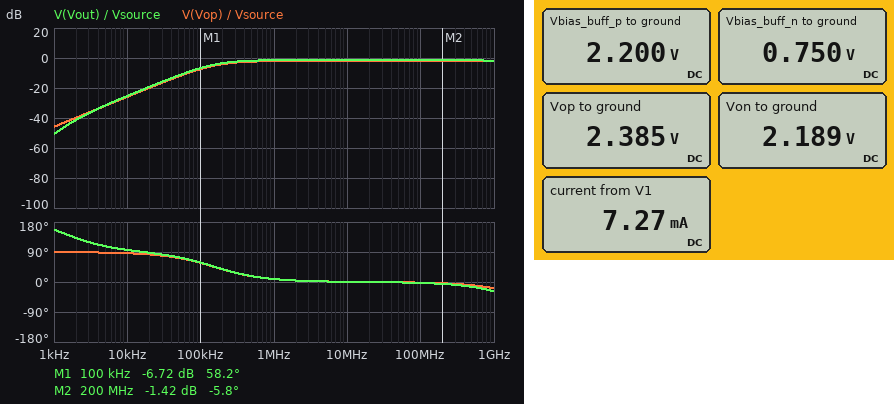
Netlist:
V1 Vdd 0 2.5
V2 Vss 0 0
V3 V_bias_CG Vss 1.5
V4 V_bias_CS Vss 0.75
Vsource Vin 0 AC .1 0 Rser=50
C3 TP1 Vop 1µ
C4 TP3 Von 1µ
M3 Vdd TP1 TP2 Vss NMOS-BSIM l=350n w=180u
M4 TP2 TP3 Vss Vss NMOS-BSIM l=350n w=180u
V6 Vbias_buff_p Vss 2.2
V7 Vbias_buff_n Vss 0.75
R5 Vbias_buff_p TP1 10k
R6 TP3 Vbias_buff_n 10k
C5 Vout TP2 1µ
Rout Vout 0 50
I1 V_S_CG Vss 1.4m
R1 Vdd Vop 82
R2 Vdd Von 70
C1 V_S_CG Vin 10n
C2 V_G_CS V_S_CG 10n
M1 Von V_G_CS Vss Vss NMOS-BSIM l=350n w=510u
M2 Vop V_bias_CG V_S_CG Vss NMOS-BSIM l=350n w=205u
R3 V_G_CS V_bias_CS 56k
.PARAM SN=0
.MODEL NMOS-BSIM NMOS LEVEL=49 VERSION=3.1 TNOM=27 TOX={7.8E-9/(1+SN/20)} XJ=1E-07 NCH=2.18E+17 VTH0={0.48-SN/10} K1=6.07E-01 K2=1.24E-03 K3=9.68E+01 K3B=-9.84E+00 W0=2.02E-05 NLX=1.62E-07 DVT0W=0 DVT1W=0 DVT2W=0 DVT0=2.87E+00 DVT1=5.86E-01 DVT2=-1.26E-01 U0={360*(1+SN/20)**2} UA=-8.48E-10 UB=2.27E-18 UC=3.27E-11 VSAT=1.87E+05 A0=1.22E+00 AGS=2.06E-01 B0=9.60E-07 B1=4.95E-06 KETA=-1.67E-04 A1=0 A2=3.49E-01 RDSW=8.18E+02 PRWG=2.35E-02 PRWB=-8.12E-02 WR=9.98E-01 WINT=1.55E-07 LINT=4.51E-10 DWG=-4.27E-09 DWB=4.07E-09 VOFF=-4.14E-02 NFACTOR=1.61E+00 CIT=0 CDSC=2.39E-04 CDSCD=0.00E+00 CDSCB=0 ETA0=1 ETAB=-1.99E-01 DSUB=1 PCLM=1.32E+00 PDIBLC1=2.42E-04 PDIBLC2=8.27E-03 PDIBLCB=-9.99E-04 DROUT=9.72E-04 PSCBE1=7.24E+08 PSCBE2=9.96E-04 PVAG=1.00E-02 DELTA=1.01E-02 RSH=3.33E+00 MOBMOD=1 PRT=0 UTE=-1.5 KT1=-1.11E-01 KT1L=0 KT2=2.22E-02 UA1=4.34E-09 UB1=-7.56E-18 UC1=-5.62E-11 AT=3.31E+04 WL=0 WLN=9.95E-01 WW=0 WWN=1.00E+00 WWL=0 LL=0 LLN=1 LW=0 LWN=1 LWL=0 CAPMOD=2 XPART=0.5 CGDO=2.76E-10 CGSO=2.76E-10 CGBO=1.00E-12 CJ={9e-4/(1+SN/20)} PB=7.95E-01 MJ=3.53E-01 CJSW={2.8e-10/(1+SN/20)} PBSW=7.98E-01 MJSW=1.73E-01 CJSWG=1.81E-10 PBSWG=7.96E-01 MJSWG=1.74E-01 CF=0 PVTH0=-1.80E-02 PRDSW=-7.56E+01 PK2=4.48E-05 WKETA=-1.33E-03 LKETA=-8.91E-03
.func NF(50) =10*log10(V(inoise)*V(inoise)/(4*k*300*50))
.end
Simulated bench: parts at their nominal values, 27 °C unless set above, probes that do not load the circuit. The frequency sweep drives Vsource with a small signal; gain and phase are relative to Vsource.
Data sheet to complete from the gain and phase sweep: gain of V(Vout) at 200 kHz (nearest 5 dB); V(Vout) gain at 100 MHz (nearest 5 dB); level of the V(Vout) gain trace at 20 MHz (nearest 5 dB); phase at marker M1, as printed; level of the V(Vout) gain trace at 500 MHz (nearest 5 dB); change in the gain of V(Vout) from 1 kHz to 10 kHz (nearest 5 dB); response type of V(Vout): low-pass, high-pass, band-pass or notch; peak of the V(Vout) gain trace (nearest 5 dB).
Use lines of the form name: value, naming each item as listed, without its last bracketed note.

gain of V(Vout) at 200 kHz: -5 dB
V(Vout) gain at 100 MHz: 0 dB
level of the V(Vout) gain trace at 20 MHz: 0 dB
phase at marker M1, as printed: 58.2 deg
level of the V(Vout) gain trace at 500 MHz: 0 dB
change in the gain of V(Vout) from 1 kHz to 10 kHz: 25 dB
response type of V(Vout): low-pass, high-pass, band-pass or notch: high-pass
peak of the V(Vout) gain trace: 0 dB
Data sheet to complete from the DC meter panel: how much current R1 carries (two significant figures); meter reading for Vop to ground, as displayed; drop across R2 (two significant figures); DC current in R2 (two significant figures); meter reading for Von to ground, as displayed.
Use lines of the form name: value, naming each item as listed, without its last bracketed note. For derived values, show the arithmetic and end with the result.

how much current R1 carries: (2.5 V - 2.385 V) / 82 Ω = 1.4 mA
meter reading for Vop to ground, as displayed: 2.385 V
drop across R2: 2.5 V - 2.189 V = 310 mV
DC current in R2: (2.5 V - 2.189 V) / 70 Ω = 4.4 mA
meter reading for Von to ground, as displayed: 2.189 V
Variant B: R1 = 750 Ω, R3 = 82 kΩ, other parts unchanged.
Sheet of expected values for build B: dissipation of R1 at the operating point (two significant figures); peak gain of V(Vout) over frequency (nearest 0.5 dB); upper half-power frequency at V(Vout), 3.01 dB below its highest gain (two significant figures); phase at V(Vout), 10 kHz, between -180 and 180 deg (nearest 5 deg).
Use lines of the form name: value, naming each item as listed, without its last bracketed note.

dissipation of R1 at the operating point: 1.5 mW
peak gain of V(Vout) over frequency: 9.5 dB
upper half-power frequency at V(Vout), 3.01 dB below its highest gain: 910 MHz
phase at V(Vout), 10 kHz, between -180 and 180 deg: 95 deg
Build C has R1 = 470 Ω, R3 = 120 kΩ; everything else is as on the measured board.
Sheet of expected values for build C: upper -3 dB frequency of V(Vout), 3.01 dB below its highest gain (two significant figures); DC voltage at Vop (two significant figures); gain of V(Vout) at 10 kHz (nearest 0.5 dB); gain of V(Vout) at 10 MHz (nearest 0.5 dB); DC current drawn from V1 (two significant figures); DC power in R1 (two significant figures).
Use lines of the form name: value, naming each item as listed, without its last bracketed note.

upper -3 dB frequency of V(Vout), 3.01 dB below its highest gain: 1.4 GHz
DC voltage at Vop: 1.8 V
gain of V(Vout) at 10 kHz: -16.5 dB
gain of V(Vout) at 10 MHz: 7.0 dB
DC current drawn from V1: 7.3 mA
DC power in R1: 920 µW
